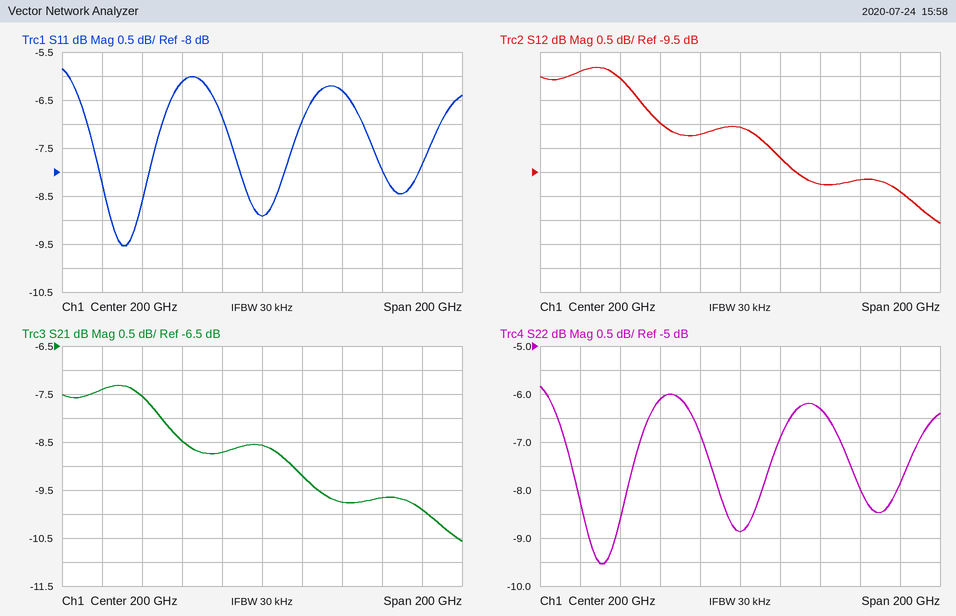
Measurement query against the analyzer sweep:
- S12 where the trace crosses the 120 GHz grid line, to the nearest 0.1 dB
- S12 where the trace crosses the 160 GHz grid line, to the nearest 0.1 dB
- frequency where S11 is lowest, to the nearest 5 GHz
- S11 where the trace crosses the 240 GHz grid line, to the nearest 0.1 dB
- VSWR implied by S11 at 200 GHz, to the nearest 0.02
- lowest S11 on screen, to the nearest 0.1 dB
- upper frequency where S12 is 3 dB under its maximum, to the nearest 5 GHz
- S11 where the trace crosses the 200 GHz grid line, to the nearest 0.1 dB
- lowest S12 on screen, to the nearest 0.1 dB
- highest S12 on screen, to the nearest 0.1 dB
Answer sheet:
-7.4 dB
-8.5 dB
130 GHz
-6.3 dB
2.12
-9.5 dB
290 GHz
-8.9 dB
-10.6 dB
-7.3 dB
